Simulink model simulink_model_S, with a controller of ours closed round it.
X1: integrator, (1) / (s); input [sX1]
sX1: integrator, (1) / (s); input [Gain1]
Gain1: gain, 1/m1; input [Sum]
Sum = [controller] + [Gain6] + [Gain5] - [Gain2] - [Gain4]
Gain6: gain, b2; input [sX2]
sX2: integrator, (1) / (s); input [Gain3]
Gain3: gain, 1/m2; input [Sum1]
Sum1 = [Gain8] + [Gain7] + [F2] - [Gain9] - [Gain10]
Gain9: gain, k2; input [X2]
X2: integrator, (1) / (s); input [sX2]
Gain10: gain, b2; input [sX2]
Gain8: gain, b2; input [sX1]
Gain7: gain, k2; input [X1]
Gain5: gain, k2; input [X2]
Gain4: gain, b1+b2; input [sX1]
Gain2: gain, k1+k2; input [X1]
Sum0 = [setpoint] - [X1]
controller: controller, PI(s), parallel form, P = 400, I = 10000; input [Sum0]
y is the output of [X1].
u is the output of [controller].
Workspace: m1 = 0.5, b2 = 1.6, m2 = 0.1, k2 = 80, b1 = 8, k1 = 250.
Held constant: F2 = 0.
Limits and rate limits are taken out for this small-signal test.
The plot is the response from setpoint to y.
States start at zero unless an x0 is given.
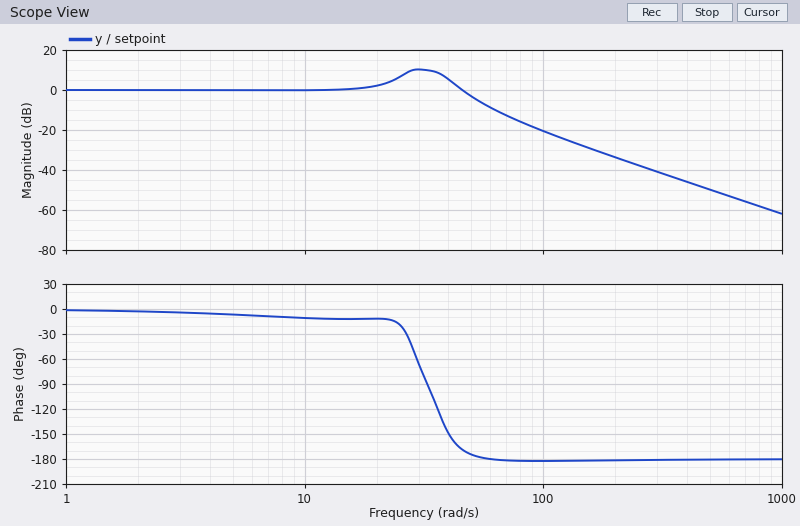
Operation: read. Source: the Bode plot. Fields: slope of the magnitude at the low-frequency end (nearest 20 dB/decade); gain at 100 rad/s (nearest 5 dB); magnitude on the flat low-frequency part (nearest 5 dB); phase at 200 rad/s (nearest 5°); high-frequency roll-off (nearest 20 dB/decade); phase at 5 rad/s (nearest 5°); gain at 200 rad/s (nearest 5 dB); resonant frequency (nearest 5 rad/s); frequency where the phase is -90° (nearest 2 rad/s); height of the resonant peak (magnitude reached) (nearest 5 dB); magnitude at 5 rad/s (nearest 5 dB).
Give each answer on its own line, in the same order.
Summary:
0 dB/decade
-20 dB
0 dB
-180°
-40 dB/decade
-5°
-35 dB
30 rad/s
32 rad/s
10 dB
0 dB
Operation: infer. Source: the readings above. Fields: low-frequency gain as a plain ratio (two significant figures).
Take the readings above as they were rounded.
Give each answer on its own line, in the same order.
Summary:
1.0
